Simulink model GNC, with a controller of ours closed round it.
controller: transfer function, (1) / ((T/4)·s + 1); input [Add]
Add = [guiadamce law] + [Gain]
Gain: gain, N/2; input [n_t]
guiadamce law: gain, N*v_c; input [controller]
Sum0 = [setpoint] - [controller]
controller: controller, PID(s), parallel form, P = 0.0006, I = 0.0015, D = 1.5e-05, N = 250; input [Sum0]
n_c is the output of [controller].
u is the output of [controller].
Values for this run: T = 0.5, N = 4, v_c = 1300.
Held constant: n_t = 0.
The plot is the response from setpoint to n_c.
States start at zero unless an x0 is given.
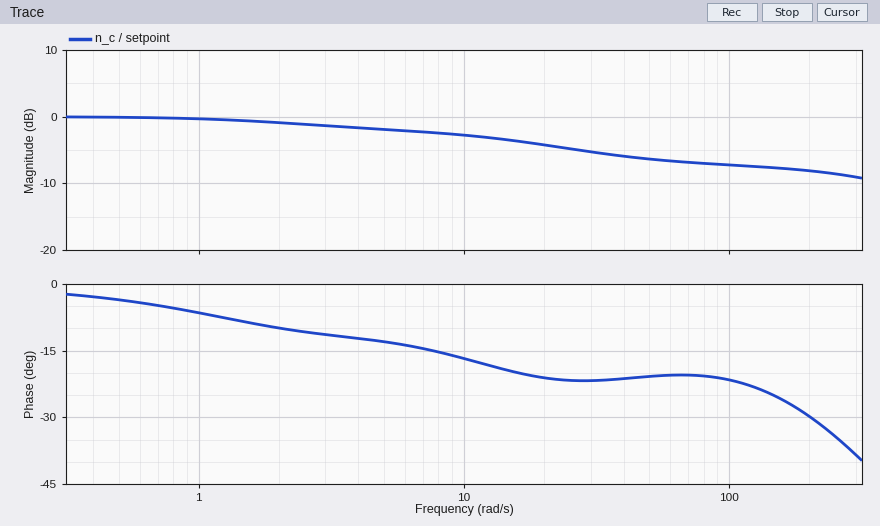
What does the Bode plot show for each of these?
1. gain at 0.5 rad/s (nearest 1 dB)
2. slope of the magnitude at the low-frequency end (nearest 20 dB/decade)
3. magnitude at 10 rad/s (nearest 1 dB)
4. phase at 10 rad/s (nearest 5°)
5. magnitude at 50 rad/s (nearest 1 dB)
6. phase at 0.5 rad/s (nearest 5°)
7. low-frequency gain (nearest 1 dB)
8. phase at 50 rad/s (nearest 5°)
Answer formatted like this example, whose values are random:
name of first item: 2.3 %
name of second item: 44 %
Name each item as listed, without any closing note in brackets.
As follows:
gain at 0.5 rad/s: 0 dB
slope of the magnitude at the low-frequency end: 0 dB/decade
magnitude at 10 rad/s: -3 dB
phase at 10 rad/s: -15°
magnitude at 50 rad/s: -6 dB
phase at 0.5 rad/s: -5°
low-frequency gain: 0 dB
phase at 50 rad/s: -20°
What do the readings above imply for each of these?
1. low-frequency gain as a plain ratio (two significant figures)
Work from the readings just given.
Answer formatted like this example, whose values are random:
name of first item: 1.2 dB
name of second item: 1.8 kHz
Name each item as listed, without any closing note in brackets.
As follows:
low-frequency gain as a plain ratio: 1.0
